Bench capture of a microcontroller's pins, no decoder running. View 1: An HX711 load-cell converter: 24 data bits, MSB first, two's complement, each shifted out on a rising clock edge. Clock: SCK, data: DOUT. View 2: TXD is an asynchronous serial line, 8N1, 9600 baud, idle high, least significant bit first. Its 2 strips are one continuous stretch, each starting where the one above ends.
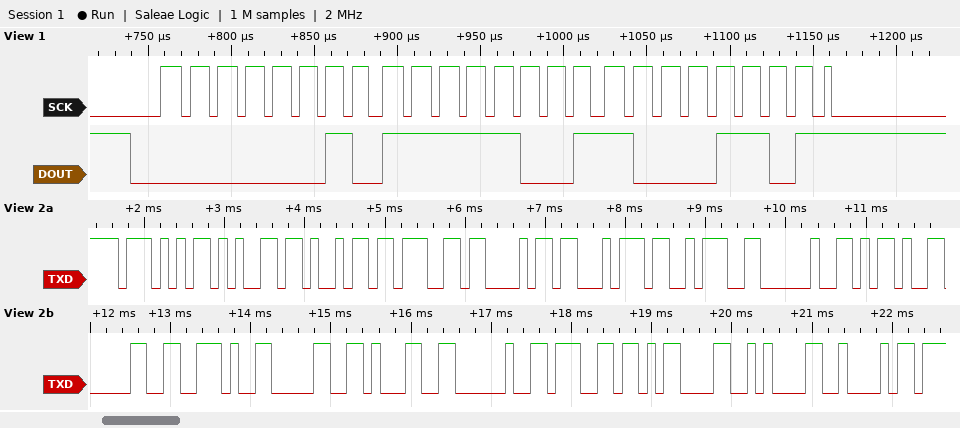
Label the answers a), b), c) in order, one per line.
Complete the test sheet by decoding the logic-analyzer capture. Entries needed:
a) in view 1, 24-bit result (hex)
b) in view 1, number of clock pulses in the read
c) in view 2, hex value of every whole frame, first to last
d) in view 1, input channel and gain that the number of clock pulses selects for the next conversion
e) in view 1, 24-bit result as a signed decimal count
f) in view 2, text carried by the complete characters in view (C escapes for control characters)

a) 0x02F98D
b) 25
c) 0x57 0x65 0x69 0x67 0x68 0x74 0x3A 0x20 0x2D 0x30 0x2E 0x30 0x31 0x20 0x67 0x0D 0x0A 0x42
d) channel A, gain 128
e) 194957
f) "Weight: -0.01 g\r\nB"
